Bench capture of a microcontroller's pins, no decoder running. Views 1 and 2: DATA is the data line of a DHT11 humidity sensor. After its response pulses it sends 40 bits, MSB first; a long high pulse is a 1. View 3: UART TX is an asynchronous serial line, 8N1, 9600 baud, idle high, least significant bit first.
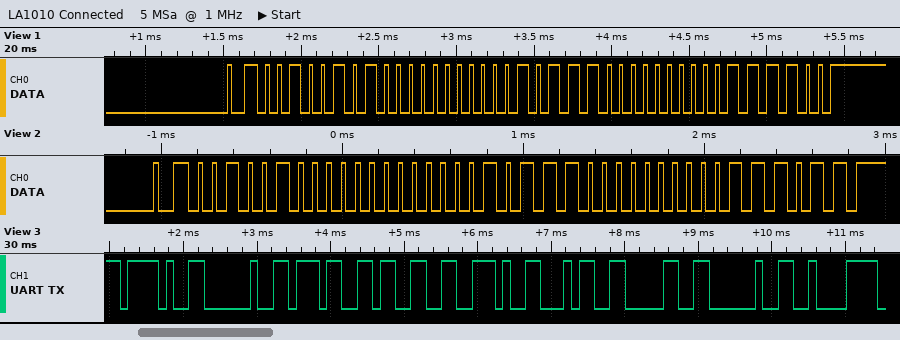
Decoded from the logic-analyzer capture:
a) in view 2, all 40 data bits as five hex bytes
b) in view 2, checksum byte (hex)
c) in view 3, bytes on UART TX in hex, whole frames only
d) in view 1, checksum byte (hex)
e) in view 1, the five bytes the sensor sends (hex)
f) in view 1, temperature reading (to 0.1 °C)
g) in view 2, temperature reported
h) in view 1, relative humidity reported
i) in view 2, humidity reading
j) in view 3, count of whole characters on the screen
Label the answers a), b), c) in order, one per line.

a) 24 00 17 00 3B
b) 0x3B
c) 0x2F 0x20 0x37 0x33 0x2E 0x34 0x30 0x20 0xC2
d) 0x3C
e) 25 00 17 00 3C
f) 23.0 °C
g) 23.0 °C
h) 37 %
i) 36 %
j) 9
